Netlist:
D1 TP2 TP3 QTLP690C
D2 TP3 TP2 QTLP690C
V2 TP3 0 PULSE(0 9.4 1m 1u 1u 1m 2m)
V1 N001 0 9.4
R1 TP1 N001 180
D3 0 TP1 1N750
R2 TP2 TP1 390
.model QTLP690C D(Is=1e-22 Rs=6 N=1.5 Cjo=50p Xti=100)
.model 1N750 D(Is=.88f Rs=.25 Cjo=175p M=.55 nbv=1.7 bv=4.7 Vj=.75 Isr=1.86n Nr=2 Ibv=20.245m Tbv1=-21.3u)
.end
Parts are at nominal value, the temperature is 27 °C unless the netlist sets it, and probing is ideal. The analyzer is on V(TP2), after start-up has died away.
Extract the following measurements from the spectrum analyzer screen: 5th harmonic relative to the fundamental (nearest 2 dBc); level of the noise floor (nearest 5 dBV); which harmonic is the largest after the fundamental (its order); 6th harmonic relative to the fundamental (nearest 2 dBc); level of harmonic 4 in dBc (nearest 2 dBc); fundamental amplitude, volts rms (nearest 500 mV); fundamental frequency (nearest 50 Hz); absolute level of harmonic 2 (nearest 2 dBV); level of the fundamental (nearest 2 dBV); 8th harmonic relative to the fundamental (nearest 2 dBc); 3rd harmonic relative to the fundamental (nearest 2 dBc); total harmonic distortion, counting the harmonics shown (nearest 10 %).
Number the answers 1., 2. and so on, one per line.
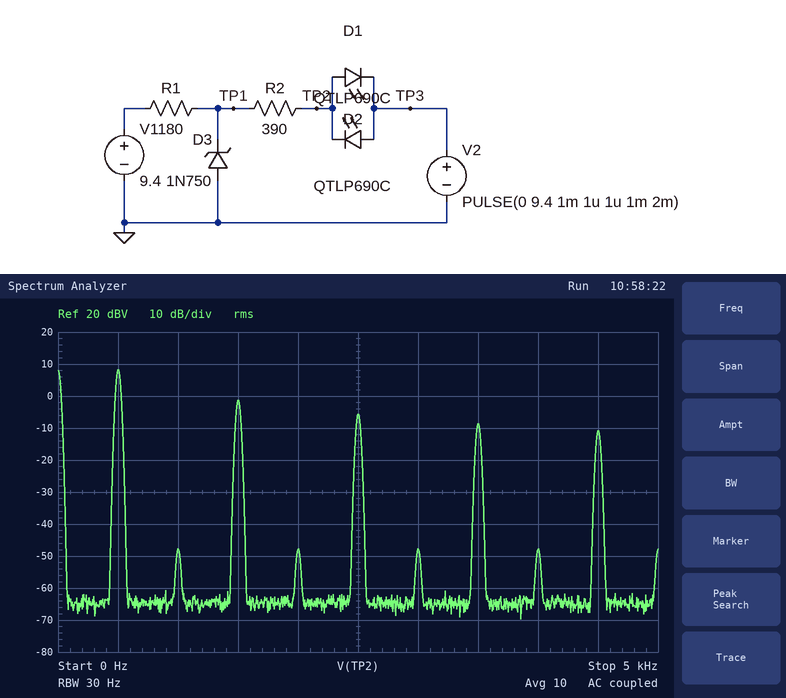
1. -14 dBc
2. -65 dBV
3. 3
4. -56 dBc
5. -56 dBc
6. 2.5 V
7. 500 Hz
8. -48 dBV
9. 8 dBV
10. -56 dBc
11. -10 dBc
12. 40 %
